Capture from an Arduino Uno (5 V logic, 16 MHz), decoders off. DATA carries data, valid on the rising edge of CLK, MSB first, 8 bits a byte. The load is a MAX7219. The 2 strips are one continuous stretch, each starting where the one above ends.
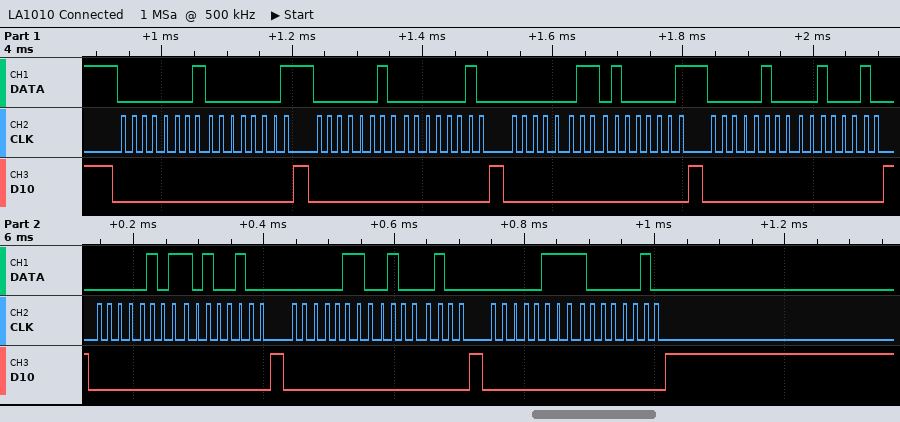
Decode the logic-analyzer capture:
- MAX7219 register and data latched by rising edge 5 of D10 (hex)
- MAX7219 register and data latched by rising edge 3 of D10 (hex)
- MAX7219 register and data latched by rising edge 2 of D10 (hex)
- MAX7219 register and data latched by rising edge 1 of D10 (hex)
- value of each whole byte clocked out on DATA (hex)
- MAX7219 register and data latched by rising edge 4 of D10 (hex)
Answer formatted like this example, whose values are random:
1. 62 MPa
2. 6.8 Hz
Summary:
1. register 0x5, data 0xA4
2. register 0x3, data 0x41
3. register 0x2, data 0x02
4. register 0x1, data 0x01
5. 0x01 0x01 0x02 0x02 0x03 0x41 0x04 0x22 0x05 0xA4 0x06 0x44 0x07 0x82
6. register 0x4, data 0x22
